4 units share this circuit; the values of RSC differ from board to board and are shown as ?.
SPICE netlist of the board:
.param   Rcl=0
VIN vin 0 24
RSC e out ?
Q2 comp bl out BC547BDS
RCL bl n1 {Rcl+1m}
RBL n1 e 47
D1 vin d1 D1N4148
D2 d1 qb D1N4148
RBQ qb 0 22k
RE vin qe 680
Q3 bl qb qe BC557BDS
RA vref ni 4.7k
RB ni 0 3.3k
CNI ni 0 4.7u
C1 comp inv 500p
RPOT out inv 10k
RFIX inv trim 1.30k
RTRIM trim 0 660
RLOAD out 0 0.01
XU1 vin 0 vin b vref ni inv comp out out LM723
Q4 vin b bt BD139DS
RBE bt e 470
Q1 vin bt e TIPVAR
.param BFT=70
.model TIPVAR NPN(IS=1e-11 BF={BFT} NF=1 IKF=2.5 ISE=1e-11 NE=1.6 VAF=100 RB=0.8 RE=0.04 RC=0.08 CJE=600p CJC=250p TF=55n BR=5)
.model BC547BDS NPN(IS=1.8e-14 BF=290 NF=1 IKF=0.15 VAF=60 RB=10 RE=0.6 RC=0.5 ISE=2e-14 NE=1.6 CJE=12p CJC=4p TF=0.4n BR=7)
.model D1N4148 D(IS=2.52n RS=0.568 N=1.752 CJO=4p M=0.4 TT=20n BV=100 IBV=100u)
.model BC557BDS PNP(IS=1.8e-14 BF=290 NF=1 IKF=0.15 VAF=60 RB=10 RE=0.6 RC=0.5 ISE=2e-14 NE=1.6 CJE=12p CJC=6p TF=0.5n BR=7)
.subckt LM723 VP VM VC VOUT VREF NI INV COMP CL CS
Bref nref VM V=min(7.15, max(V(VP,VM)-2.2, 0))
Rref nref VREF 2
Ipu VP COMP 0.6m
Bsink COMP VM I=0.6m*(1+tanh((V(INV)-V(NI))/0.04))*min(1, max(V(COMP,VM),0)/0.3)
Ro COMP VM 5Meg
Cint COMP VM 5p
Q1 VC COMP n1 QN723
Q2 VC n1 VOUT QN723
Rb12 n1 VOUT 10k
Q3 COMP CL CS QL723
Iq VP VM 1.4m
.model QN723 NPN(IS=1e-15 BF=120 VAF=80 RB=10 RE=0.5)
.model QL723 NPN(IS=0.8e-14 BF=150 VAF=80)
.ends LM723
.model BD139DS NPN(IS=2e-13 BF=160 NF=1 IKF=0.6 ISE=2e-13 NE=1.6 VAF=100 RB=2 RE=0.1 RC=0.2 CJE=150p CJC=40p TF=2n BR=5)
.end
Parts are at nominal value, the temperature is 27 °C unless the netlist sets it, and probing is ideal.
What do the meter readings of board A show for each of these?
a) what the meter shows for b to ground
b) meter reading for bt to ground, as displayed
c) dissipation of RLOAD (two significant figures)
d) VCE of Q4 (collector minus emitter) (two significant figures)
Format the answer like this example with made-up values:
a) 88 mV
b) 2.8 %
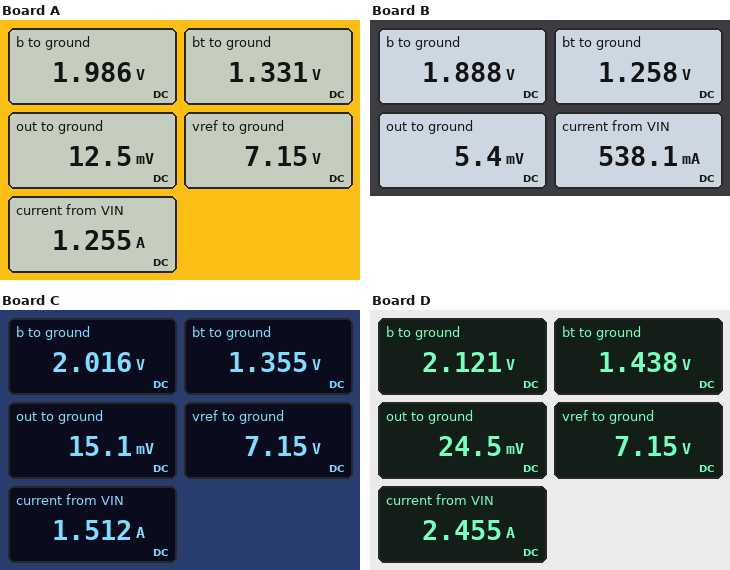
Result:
a) 1.986 V
b) 1.331 V
c) 16 mW
d) 23 V
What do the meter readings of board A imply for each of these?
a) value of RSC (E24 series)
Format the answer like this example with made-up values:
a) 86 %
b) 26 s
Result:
a) 0.47 Ω
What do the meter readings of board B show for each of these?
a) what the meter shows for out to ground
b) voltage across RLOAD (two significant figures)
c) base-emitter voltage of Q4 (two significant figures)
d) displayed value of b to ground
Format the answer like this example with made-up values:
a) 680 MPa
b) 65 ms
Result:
a) 5.4 mV
b) 5.4 mV
c) 630 mV
d) 1.888 V
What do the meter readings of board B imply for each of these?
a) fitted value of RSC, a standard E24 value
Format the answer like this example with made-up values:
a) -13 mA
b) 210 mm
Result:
a) 1.1 Ω
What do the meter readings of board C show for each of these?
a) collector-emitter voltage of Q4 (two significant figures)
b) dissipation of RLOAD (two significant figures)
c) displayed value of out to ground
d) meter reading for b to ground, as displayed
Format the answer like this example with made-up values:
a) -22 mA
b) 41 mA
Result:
a) 23 V
b) 23 mW
c) 15.1 mV
d) 2.016 V
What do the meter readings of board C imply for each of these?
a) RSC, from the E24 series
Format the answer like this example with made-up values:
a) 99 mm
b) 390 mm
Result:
a) 0.39 Ω
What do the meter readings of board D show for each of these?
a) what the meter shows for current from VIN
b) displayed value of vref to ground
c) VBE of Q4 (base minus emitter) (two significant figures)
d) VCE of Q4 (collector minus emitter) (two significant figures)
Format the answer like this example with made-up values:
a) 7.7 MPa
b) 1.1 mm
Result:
a) 2.455 A
b) 7.15 V
c) 680 mV
d) 23 V
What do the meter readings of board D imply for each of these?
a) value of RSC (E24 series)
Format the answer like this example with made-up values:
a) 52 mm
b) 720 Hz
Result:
a) 0.24 Ω
